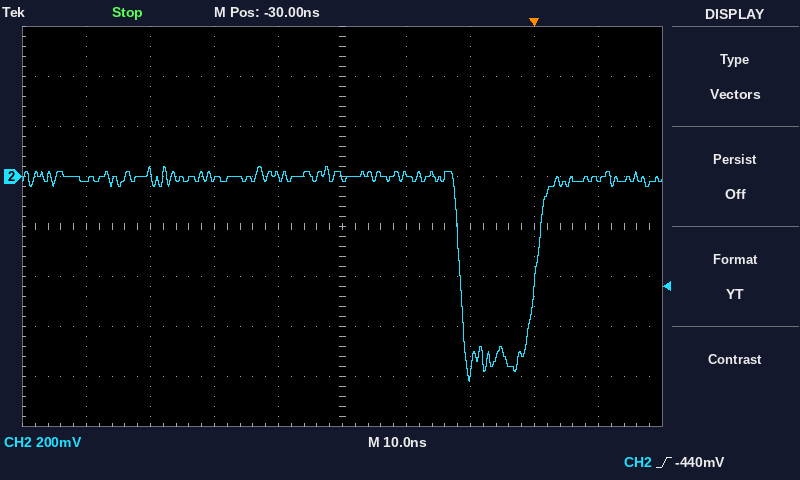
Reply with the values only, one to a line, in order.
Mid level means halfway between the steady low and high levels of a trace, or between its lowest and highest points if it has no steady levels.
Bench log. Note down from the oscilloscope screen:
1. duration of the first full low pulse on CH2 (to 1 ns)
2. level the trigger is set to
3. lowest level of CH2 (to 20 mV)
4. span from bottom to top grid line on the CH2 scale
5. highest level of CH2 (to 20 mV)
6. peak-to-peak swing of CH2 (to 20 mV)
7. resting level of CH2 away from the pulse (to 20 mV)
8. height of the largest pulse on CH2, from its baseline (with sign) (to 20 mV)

12 ns
-440 mV
-820 mV
1.6 V
40 mV
860 mV
0 mV
-820 mV
